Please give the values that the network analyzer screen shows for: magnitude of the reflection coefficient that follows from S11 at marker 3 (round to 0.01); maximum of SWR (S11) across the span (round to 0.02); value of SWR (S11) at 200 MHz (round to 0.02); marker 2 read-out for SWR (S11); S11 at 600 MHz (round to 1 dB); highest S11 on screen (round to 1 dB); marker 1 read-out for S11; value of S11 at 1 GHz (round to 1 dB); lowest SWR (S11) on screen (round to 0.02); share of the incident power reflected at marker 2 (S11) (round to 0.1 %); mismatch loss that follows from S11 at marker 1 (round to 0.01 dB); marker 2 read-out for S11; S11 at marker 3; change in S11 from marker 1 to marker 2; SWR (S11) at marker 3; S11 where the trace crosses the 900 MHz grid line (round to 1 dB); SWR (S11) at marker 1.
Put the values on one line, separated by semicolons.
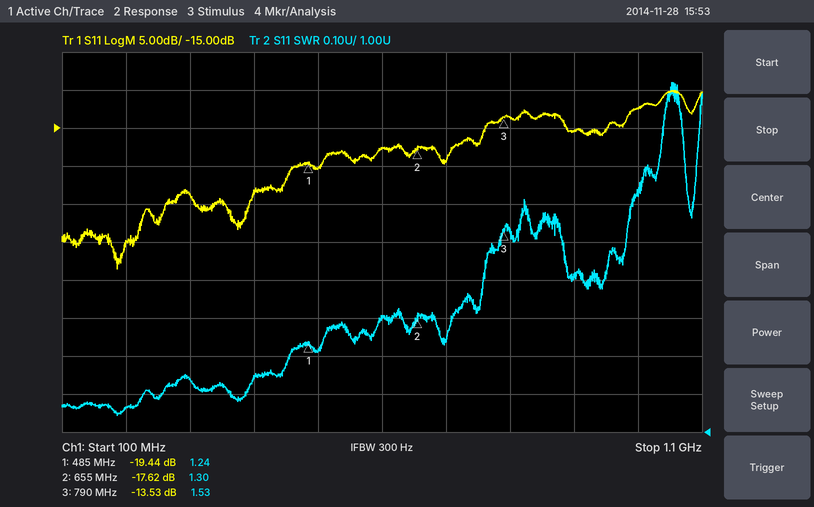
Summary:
0.21; 1.92; 1.06; 1.30; -18 dB; -10 dB; -19.44 dB; -12 dB; 1.04; 1.7 %; 0.05 dB; -17.62 dB; -13.53 dB; 1.82 dB; 1.53; -15 dB; 1.24
